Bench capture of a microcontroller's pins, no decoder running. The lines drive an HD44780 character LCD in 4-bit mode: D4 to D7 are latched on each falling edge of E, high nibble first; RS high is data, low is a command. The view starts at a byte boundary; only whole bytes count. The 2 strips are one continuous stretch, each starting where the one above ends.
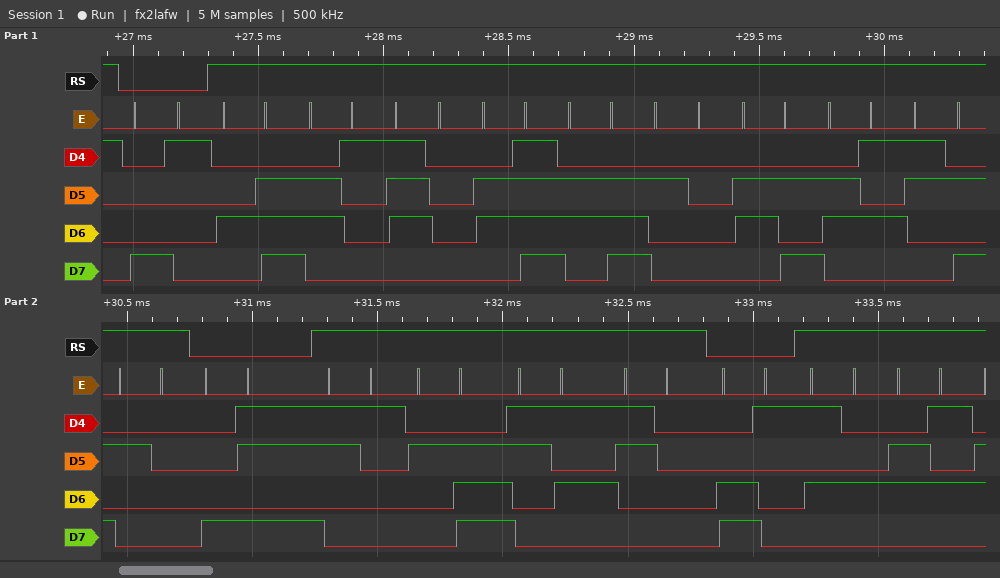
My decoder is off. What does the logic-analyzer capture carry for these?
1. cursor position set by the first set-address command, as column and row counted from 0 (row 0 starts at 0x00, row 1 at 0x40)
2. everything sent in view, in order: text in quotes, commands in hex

column 1, row 0
0x81 "Napon je: " 0x8B "1.50" 0xC1 "Te"
